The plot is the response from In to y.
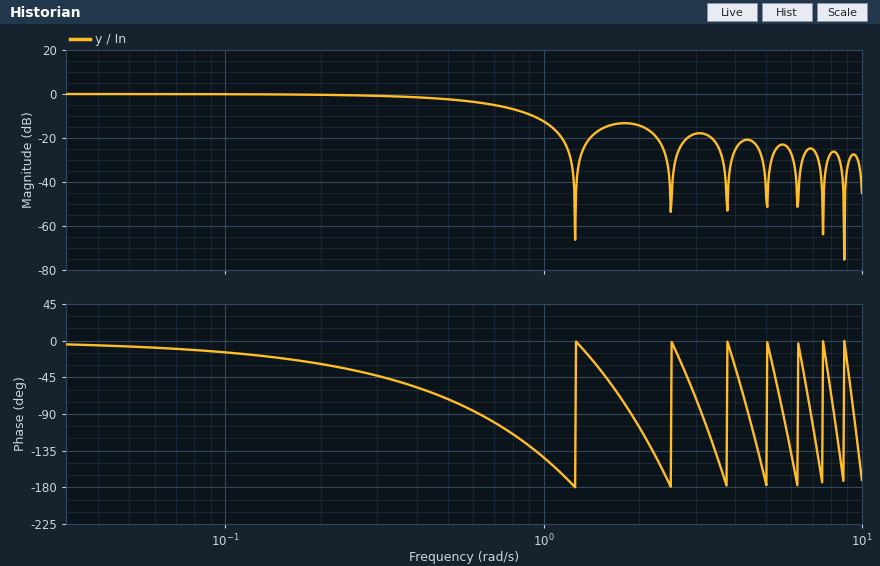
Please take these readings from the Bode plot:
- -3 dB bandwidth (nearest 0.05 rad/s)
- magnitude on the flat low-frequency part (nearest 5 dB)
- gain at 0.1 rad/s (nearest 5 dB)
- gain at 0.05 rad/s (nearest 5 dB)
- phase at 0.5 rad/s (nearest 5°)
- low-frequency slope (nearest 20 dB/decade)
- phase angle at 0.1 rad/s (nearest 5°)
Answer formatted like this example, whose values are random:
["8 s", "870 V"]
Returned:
["0.55 rad/s", "0 dB", "0 dB", "0 dB", "-70°", "0 dB/decade", "-15°"]
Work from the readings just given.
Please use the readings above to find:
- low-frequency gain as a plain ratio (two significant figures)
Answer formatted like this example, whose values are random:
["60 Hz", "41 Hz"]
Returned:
["1.0"]
